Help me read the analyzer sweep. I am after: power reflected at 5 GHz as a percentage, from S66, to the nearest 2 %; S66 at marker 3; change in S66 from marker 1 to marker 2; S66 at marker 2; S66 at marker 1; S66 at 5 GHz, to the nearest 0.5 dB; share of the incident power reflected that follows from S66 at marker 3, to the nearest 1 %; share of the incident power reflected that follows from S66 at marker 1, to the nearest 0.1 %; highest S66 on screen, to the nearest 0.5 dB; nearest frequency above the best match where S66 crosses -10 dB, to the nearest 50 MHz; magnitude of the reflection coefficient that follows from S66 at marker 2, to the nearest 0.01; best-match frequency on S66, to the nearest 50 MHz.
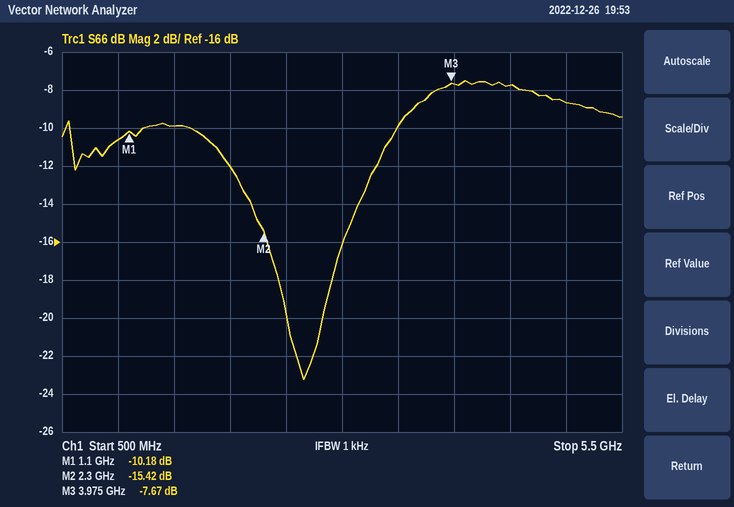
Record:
14 %
-7.67 dB
-5.24 dB
-15.42 dB
-10.18 dB
-8.5 dB
17 %
9.6 %
-7.5 dB
3.50 GHz
0.17
2.65 GHz
